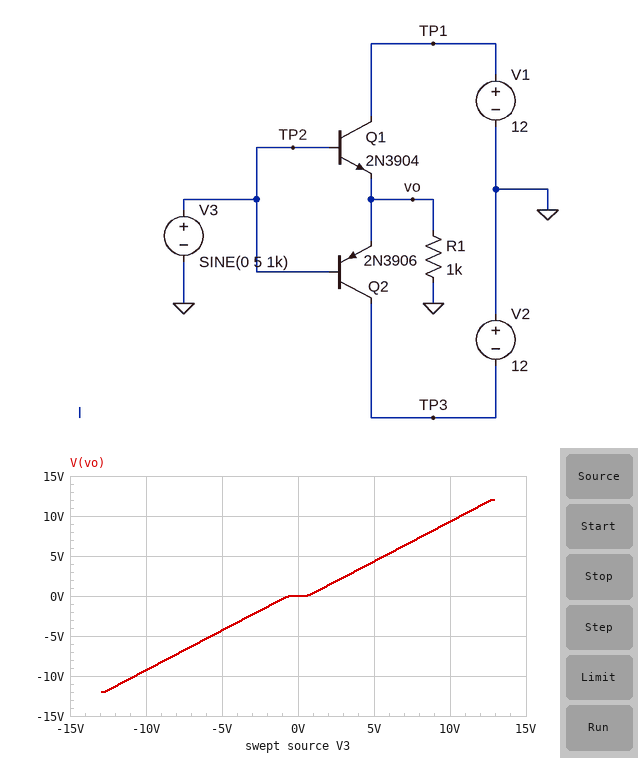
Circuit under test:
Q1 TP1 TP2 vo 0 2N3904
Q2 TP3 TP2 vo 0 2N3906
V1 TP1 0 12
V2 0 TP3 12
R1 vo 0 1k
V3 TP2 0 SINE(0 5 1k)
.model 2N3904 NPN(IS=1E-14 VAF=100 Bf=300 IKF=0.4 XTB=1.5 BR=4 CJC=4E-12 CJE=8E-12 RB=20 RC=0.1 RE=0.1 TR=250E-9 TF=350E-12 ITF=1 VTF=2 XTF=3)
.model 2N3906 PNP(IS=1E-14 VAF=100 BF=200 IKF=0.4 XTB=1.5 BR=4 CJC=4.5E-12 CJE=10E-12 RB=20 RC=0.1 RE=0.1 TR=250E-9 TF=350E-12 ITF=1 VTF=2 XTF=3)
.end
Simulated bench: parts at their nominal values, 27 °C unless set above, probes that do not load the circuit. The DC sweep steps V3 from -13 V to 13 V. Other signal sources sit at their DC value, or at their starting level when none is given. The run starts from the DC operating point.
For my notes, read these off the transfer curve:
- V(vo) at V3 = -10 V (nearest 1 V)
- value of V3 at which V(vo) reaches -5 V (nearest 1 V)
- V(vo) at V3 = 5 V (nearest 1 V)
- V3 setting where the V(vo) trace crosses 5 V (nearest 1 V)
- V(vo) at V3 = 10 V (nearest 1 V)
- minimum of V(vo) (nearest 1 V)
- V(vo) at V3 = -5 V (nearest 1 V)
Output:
-9 V
-6 V
4 V
6 V
9 V
-12 V
-4 V
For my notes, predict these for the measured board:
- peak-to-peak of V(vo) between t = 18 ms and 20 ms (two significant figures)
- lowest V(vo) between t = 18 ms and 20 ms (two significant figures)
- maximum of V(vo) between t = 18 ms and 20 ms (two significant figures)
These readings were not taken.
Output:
8.6 V
-4.3 V
4.3 V
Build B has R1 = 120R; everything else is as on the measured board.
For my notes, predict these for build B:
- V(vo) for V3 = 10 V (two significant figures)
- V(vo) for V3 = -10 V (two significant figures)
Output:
9.2 V
-9.2 V
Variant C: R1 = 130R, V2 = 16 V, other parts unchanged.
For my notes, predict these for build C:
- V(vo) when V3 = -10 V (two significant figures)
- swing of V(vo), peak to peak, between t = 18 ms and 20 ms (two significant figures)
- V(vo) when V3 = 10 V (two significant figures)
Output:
-9.2 V
8.5 V
9.2 V
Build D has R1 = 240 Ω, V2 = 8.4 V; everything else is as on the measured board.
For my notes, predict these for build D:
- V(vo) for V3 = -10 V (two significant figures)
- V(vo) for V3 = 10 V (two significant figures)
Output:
-8.4 V
9.2 V
